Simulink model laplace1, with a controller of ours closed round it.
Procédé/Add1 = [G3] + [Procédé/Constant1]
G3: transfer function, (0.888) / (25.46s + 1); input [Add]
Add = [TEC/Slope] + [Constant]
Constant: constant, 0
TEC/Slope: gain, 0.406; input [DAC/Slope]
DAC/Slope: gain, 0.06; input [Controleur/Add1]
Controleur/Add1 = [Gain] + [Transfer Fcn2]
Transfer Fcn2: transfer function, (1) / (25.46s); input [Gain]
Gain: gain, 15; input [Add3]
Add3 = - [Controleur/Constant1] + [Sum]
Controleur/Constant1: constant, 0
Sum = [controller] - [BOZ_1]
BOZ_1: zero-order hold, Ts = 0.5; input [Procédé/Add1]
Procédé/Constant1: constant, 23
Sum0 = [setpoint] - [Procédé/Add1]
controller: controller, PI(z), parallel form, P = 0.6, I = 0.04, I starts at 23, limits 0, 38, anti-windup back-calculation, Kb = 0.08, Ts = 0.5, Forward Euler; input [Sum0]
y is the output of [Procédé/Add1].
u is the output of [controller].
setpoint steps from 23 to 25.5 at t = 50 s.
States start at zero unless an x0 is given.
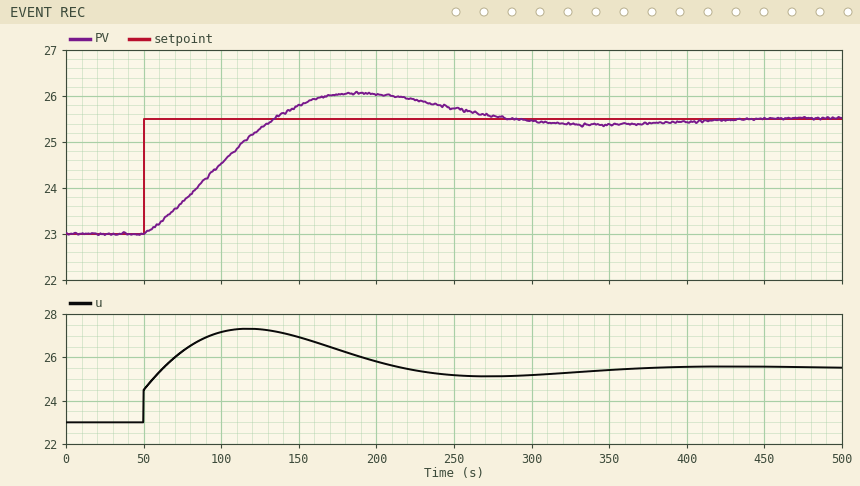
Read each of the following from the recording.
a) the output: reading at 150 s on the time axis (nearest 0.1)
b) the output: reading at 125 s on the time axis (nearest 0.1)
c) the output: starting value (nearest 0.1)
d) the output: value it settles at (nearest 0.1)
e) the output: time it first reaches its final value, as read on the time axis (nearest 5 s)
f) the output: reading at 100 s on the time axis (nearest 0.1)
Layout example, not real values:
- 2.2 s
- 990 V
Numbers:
- 25.8
- 25.3
- 23.0
- 25.5
- 135 s
- 24.5
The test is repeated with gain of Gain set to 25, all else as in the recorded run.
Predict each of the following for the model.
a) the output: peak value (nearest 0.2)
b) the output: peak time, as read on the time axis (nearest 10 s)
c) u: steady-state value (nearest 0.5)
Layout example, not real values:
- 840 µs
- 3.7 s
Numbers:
- 25.8
- 160 s
- 25.5
